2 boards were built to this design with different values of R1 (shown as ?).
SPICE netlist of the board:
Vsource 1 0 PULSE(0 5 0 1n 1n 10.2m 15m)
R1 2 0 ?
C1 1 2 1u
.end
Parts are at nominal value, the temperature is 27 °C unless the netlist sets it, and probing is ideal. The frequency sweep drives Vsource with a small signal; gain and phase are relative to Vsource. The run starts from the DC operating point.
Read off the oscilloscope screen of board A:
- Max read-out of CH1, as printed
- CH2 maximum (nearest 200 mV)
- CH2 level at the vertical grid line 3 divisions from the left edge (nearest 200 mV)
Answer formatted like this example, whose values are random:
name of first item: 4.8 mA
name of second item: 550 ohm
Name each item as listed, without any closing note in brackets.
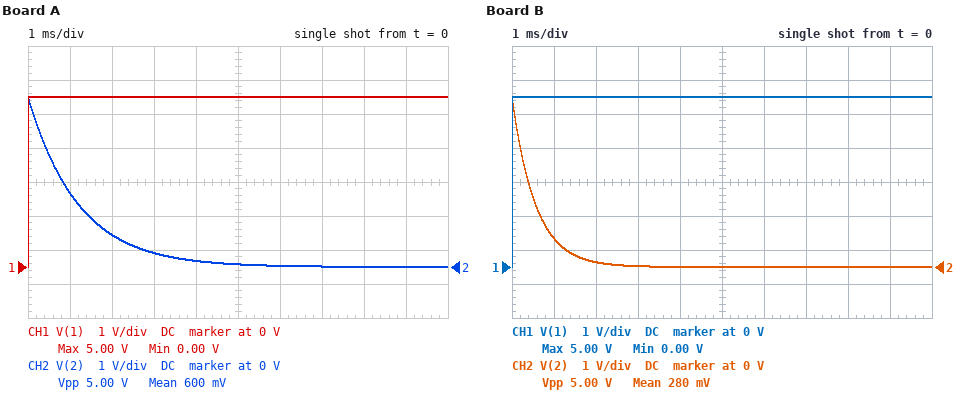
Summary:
Max read-out of CH1, as printed: 5.00 V
CH2 maximum: 5.0 V
CH2 level at the vertical grid line 3 divisions from the left edge: 400 mV
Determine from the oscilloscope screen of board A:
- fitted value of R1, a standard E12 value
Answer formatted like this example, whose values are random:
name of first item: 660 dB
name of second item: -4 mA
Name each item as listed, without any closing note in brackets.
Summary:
fitted value of R1, a standard E12 value: 1.2 kΩ
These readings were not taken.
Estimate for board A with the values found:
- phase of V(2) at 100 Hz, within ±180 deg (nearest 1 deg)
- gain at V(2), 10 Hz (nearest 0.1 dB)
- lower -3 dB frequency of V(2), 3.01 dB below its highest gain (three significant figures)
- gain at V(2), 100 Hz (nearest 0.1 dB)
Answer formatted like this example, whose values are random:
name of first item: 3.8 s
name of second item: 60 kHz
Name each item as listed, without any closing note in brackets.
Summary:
phase of V(2) at 100 Hz, within ±180 deg: 53 deg
gain at V(2), 10 Hz: -22.5 dB
lower -3 dB frequency of V(2), 3.01 dB below its highest gain: 133 Hz
gain at V(2), 100 Hz: -4.4 dB
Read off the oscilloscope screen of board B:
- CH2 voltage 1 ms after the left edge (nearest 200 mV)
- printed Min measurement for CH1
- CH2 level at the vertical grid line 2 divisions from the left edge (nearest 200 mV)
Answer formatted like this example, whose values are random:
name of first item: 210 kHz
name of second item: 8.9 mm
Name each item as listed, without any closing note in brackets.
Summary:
CH2 voltage 1 ms after the left edge: 800 mV
printed Min measurement for CH1: 0.00 V
CH2 level at the vertical grid line 2 divisions from the left edge: 200 mV
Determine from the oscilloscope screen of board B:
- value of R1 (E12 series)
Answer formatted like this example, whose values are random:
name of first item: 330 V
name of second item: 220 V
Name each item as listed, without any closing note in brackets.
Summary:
value of R1: 560 Ω
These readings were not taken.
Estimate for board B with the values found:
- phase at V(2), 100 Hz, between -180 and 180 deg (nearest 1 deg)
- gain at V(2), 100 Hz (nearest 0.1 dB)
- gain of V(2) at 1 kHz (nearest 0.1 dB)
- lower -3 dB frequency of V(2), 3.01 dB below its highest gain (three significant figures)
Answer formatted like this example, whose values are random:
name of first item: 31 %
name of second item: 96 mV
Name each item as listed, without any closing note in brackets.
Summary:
phase at V(2), 100 Hz, between -180 and 180 deg: 71 deg
gain at V(2), 100 Hz: -9.6 dB
gain of V(2) at 1 kHz: -0.3 dB
lower -3 dB frequency of V(2), 3.01 dB below its highest gain: 284 Hz
